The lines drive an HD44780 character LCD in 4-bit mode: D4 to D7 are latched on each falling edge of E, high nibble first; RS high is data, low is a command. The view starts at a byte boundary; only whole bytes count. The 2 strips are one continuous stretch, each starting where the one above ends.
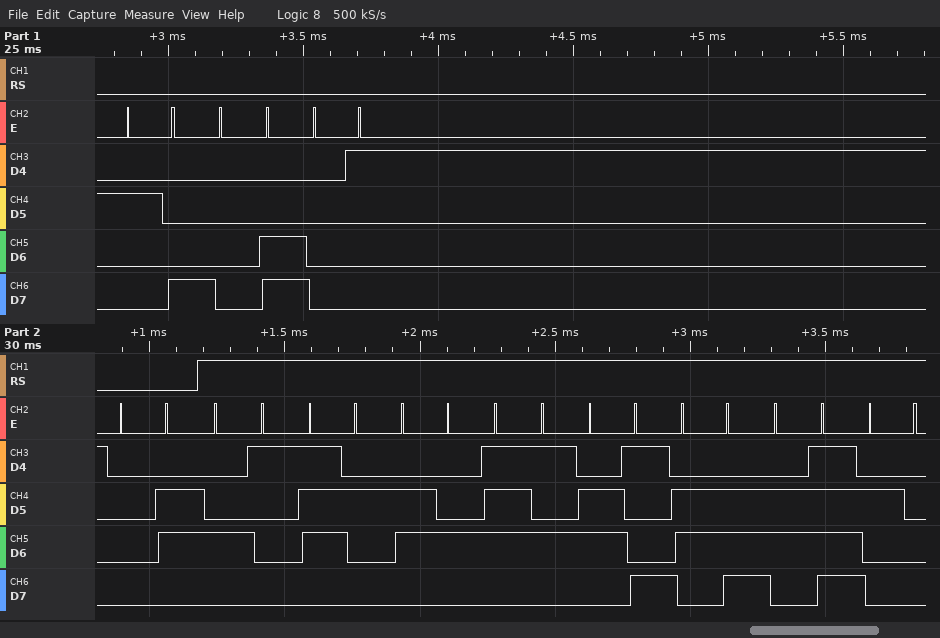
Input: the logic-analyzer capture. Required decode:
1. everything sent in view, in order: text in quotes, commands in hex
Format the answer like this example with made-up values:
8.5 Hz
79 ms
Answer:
0x28 0x0C 0x01 0x06 "Arduino "
